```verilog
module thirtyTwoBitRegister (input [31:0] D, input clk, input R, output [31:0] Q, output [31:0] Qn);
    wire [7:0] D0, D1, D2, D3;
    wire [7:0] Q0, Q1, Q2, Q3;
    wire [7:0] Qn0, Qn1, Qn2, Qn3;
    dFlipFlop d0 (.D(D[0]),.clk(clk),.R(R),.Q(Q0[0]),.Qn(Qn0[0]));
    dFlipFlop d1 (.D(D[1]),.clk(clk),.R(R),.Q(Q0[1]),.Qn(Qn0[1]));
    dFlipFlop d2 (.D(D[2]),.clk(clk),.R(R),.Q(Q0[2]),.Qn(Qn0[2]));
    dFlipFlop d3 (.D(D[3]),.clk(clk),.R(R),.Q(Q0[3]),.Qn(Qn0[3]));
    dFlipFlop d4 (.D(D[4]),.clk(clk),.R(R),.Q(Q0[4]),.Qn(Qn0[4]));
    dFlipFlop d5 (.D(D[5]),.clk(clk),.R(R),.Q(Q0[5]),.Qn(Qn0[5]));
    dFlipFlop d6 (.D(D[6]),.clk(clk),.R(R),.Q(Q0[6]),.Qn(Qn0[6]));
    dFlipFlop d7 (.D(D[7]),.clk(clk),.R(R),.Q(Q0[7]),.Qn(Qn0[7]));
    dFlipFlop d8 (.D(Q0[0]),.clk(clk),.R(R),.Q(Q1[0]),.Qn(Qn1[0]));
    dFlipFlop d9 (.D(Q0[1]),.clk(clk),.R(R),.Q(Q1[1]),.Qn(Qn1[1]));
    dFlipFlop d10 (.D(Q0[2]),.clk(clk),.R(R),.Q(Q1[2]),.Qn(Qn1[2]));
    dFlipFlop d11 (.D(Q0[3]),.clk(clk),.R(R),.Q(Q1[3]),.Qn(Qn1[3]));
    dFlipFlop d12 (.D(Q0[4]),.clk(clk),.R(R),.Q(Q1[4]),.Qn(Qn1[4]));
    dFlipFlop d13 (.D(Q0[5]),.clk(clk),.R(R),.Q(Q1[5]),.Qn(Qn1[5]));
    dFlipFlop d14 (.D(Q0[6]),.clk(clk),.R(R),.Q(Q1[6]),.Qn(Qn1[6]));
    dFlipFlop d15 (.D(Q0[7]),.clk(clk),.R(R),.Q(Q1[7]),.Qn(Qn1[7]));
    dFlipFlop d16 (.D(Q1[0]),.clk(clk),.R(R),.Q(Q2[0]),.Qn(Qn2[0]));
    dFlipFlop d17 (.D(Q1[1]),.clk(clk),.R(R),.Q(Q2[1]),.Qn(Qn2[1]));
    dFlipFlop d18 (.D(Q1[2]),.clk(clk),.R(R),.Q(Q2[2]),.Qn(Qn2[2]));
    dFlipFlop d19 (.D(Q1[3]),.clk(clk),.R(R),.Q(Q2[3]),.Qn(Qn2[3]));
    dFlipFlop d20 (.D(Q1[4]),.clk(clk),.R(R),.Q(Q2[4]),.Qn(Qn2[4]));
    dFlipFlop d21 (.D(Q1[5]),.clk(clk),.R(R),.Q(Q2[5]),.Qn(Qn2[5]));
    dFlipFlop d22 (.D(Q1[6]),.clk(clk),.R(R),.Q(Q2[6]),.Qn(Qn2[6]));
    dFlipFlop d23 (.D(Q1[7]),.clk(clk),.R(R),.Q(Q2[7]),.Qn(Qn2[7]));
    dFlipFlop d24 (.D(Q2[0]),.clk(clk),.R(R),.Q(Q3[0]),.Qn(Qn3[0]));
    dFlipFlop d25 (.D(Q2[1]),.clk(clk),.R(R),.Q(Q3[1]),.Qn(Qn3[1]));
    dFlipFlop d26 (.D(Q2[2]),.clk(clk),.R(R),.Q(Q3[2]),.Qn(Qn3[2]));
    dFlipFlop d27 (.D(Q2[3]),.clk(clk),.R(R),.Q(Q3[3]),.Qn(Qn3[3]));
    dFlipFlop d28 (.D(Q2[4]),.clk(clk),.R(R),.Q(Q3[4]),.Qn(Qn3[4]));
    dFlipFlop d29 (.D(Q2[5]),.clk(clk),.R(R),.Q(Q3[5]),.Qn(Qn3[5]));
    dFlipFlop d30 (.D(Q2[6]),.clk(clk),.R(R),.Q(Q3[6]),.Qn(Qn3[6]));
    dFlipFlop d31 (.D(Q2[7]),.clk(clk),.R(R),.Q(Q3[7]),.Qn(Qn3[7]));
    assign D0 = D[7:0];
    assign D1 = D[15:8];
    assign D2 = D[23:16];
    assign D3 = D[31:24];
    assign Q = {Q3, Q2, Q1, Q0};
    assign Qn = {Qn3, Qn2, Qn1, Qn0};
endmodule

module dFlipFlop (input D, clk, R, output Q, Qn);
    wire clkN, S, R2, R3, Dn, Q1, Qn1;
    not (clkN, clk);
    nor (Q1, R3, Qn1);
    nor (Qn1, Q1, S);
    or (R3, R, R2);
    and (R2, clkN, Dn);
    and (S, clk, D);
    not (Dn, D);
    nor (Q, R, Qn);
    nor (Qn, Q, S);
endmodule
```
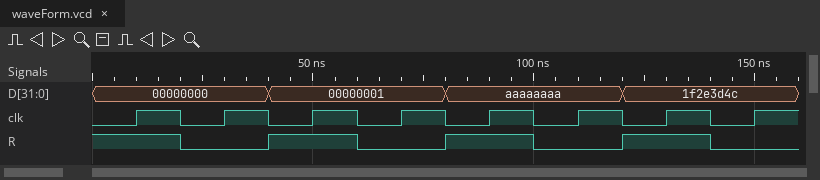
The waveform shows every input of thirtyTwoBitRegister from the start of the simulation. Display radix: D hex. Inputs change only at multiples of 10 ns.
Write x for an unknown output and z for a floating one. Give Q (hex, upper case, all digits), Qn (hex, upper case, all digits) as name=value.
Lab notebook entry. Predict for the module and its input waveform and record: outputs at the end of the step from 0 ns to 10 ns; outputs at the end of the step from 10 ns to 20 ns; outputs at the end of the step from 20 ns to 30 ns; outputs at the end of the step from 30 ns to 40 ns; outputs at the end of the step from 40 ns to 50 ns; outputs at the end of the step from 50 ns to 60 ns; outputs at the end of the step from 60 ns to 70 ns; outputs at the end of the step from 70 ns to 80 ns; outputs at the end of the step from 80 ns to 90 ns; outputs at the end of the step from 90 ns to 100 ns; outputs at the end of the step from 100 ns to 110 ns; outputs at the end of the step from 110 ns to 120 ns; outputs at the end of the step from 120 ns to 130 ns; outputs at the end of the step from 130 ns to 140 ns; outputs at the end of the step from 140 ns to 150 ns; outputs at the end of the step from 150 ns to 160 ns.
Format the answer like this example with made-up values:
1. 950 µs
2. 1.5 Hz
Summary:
1. Q=00000000, Qn=FFFFFFFF
2. Q=00000000, Qn=FFFFFFFF
3. Q=00000000, Qn=FFFFFFFF
4. Q=00000000, Qn=FFFFFFFF
5. Q=00000000, Qn=FFFFFFFF
6. Q=00000000, Qn=FFFFFFFE
7. Q=00000001, Qn=FFFFFFFE
8. Q=01010101, Qn=FEFEFEFE
9. Q=00000000, Qn=FFFFFFFF
10. Q=00000000, Qn=FFFFFF55
11. Q=000000AA, Qn=FFFFFF55
12. Q=AAAAAAAA, Qn=55555555
13. Q=00000000, Qn=FFFFFFFF
14. Q=00000000, Qn=FFFFFFB3
15. Q=0000004C, Qn=FFFFFFB3
16. Q=4C4C4C4C, Qn=B3B3B3B3
